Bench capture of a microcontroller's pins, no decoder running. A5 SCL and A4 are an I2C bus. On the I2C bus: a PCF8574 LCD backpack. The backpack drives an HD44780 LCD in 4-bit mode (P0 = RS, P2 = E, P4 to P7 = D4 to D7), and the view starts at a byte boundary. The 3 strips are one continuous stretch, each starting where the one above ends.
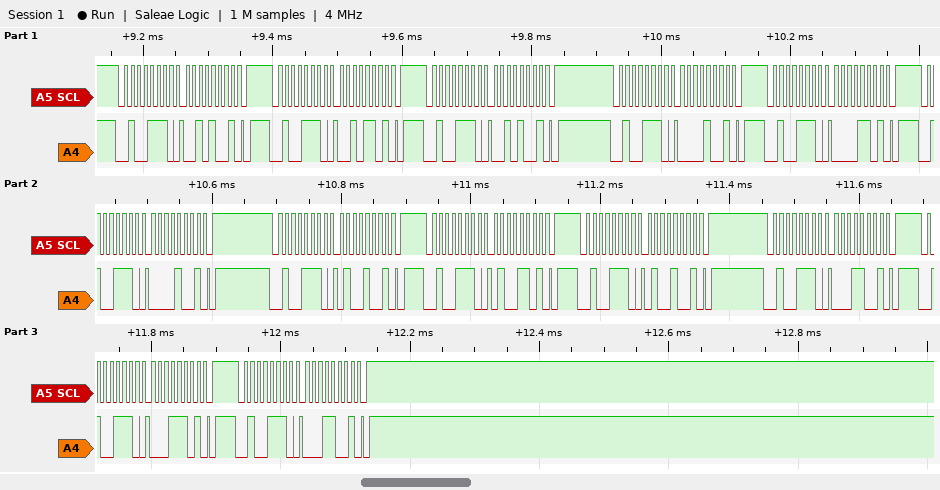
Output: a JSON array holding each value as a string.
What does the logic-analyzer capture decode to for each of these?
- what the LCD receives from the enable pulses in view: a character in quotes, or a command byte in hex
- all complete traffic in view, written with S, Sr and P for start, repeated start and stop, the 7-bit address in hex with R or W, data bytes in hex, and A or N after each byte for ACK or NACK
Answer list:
["' ' 'A'", "S 27W A 29 A P S 27W A 2D A P S 27W A 29 A P S 27W A 09 A P S 27W A 0D A P S 27W A 09 A P S 27W A 49 A P S 27W A 4D A P S 27W A 49 A P S 27W A 19 A P S 27W A 1D A P S 27W A 19 A P"]
